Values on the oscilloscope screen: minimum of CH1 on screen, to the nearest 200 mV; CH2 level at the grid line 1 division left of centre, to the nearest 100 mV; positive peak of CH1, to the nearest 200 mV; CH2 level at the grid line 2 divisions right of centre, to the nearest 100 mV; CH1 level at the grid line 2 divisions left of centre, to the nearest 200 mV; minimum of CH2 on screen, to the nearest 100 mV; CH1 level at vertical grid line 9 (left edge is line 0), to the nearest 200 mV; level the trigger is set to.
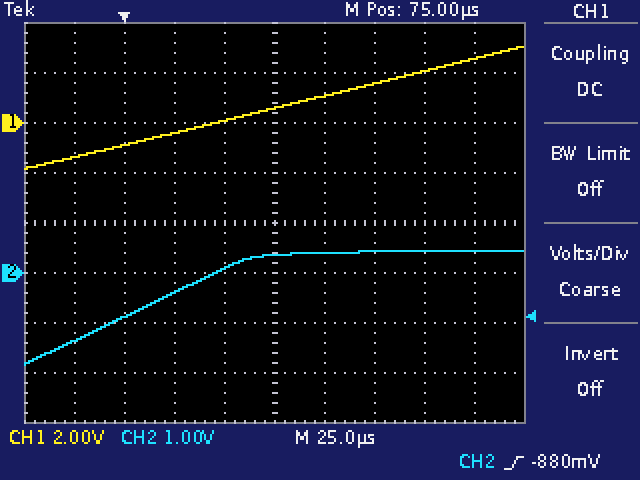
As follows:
-1.8 V
100 mV
3.0 V
400 mV
-400 mV
-1.8 V
2.6 V
-880 mV
